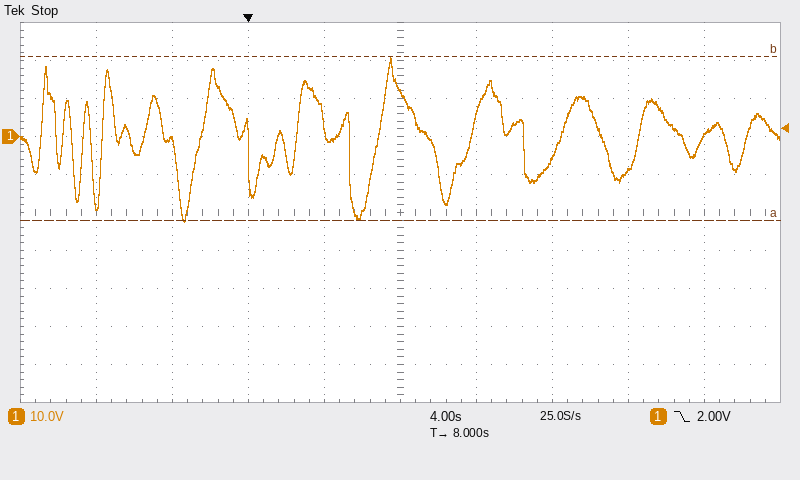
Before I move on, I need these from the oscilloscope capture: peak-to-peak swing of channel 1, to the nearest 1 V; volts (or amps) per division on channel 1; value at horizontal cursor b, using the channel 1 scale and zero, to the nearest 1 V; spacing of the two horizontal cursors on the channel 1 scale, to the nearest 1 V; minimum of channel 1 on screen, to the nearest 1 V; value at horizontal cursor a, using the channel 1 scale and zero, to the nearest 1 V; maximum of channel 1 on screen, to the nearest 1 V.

43 V
10 V
21 V
43 V
-22 V
-22 V
21 V
